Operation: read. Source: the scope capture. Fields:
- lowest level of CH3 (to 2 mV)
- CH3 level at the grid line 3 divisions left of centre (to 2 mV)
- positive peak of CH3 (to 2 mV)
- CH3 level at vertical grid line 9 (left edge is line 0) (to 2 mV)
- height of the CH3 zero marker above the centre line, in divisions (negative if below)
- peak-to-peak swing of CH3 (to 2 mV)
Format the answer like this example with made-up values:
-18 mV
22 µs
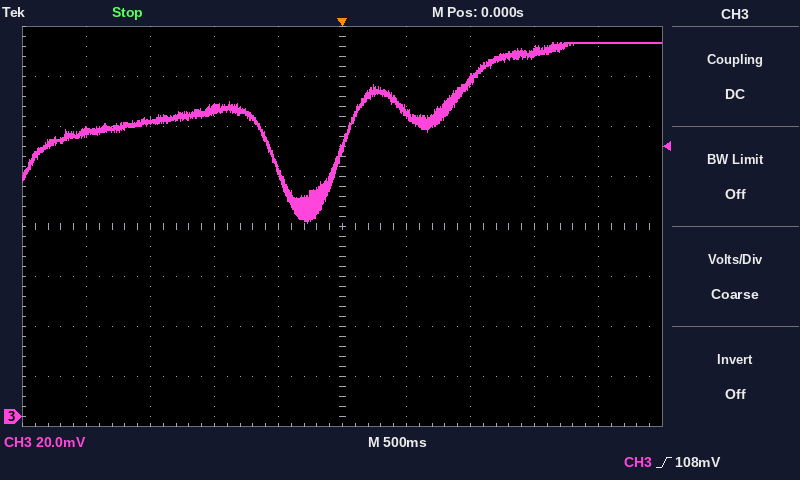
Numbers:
78 mV
118 mV
150 mV
150 mV
-3.8 div
72 mV
